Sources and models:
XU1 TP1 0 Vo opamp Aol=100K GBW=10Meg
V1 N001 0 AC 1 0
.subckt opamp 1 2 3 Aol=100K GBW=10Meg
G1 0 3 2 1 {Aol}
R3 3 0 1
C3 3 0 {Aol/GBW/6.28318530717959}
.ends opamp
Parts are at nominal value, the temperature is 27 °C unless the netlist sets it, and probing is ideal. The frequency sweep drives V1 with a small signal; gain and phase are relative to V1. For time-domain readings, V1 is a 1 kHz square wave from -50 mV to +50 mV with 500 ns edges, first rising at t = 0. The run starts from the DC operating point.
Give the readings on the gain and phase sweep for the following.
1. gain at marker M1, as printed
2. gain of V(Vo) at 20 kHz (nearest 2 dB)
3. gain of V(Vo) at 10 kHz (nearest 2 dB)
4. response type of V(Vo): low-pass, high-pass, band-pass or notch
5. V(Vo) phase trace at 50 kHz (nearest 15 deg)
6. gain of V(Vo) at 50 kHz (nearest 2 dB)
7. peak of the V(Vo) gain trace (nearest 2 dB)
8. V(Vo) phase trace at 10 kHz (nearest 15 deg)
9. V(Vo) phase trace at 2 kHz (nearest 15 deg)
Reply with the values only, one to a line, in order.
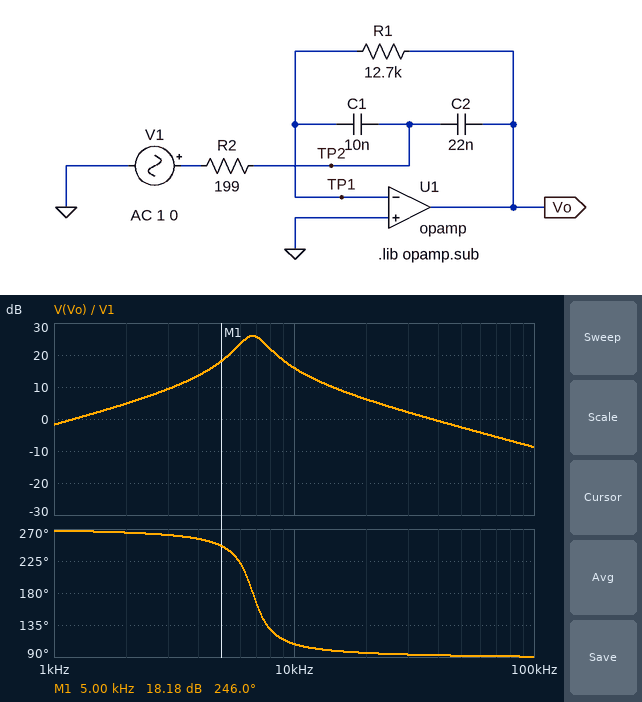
18.18 dB
6 dB
16 dB
band-pass
90 deg
-2 dB
26 dB
105 deg
270 deg
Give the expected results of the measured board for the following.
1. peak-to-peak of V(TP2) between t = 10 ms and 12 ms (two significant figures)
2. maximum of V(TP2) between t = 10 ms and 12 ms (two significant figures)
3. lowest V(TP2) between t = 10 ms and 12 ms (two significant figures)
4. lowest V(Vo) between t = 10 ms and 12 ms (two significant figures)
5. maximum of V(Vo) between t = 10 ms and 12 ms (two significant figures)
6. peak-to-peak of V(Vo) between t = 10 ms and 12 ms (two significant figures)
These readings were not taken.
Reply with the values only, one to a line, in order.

230 mV
120 mV
-120 mV
-450 mV
450 mV
900 mV
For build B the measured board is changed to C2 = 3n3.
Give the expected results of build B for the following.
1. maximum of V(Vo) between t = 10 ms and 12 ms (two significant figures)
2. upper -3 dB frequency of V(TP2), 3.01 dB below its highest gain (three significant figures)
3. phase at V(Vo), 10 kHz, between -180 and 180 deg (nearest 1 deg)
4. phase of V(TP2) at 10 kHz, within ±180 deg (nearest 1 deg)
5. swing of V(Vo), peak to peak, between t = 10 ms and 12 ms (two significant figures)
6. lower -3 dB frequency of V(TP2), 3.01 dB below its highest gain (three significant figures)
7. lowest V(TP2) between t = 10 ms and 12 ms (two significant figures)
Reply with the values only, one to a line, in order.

1.1 V
19.2 kHz
-104 deg
-14 deg
2.2 V
14.1 kHz
-110 mV
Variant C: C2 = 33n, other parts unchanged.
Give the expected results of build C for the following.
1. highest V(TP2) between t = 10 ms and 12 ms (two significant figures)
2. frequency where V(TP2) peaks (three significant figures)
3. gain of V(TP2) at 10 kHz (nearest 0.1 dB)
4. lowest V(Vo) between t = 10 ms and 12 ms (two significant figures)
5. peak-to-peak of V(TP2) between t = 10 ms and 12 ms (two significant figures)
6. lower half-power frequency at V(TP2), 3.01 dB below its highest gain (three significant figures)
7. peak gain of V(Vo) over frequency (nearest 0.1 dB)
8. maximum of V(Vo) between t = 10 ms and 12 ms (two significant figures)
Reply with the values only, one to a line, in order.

110 mV
5.38 kHz
-7.5 dB
-360 mV
230 mV
4.48 kHz
23.4 dB
360 mV
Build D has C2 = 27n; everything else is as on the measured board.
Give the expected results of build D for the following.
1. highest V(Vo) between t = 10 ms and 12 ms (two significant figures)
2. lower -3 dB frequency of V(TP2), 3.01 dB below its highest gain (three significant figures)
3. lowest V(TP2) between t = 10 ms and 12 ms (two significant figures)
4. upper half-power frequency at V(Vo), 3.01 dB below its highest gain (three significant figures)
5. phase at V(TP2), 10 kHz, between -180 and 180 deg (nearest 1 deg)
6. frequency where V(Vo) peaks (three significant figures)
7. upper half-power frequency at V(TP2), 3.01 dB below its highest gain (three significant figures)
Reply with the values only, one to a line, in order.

370 mV
5.02 kHz
-110 mV
7.00 kHz
-165 deg
6.08 kHz
6.77 kHz
